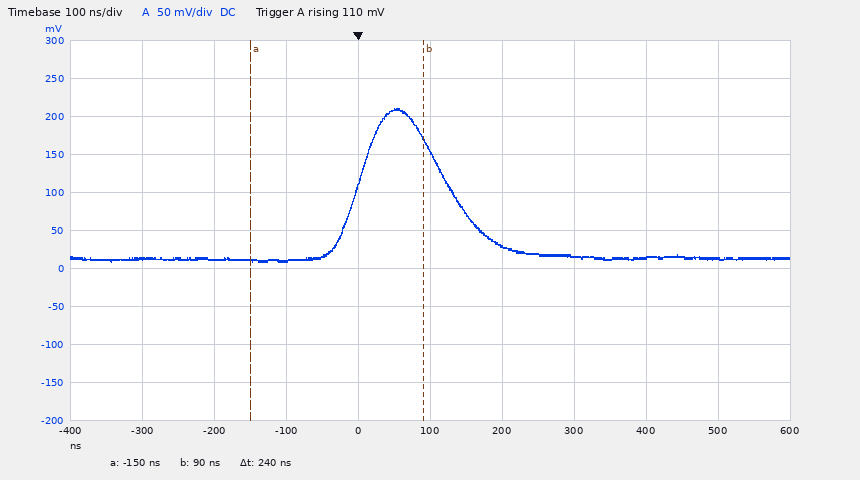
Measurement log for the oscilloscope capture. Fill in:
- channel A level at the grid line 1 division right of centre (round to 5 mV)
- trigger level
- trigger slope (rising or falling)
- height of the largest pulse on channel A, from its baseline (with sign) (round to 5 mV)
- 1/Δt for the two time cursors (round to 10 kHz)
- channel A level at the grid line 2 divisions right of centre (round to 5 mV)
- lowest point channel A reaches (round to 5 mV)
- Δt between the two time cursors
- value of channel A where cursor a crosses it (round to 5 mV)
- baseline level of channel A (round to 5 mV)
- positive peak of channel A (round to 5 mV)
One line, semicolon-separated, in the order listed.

30 mV; 110 mV; rising; +195 mV; 4.17 MHz; 15 mV; 10 mV; 240 ns; 10 mV; 15 mV; 210 mV
